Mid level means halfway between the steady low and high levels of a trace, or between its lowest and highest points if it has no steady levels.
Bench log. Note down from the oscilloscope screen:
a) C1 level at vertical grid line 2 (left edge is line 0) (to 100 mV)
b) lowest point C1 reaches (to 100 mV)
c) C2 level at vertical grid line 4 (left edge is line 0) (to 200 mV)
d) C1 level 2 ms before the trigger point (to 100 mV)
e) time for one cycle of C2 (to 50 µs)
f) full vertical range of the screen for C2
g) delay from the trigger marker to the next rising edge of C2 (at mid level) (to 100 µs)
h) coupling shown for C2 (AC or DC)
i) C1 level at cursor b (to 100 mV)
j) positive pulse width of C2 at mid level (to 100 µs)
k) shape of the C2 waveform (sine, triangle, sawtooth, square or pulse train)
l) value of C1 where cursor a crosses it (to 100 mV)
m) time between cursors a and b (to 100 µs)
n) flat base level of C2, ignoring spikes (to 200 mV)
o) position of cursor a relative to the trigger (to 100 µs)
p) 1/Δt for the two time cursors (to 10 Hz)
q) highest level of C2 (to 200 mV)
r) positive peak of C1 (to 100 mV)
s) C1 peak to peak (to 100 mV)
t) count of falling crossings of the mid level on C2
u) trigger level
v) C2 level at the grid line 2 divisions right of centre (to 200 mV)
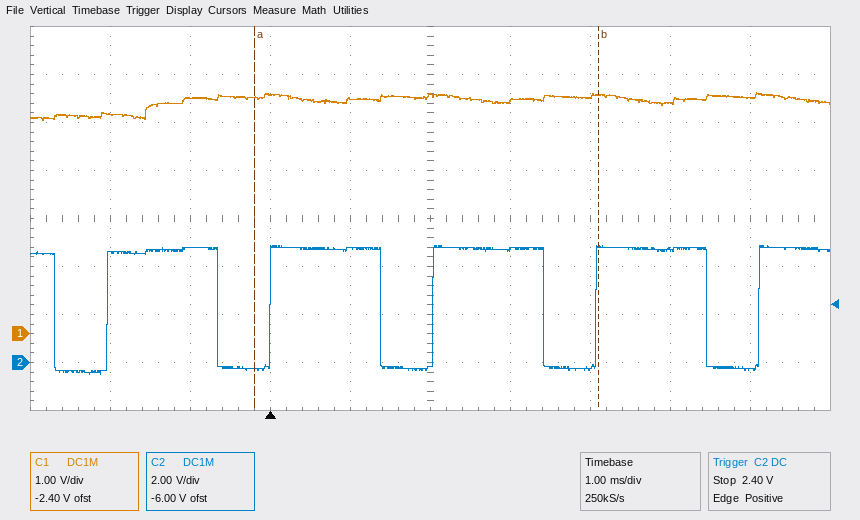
4.9 V
4.4 V
4.8 V
4.6 V
2.05 ms
16 V
2.0 ms
DC
5.0 V
1.4 ms
pulse train
4.9 V
4.3 ms
-200 mV
-200 µs
230 Hz
4.8 V
5.0 V
600 mV
5
2.40 V
-200 mV
